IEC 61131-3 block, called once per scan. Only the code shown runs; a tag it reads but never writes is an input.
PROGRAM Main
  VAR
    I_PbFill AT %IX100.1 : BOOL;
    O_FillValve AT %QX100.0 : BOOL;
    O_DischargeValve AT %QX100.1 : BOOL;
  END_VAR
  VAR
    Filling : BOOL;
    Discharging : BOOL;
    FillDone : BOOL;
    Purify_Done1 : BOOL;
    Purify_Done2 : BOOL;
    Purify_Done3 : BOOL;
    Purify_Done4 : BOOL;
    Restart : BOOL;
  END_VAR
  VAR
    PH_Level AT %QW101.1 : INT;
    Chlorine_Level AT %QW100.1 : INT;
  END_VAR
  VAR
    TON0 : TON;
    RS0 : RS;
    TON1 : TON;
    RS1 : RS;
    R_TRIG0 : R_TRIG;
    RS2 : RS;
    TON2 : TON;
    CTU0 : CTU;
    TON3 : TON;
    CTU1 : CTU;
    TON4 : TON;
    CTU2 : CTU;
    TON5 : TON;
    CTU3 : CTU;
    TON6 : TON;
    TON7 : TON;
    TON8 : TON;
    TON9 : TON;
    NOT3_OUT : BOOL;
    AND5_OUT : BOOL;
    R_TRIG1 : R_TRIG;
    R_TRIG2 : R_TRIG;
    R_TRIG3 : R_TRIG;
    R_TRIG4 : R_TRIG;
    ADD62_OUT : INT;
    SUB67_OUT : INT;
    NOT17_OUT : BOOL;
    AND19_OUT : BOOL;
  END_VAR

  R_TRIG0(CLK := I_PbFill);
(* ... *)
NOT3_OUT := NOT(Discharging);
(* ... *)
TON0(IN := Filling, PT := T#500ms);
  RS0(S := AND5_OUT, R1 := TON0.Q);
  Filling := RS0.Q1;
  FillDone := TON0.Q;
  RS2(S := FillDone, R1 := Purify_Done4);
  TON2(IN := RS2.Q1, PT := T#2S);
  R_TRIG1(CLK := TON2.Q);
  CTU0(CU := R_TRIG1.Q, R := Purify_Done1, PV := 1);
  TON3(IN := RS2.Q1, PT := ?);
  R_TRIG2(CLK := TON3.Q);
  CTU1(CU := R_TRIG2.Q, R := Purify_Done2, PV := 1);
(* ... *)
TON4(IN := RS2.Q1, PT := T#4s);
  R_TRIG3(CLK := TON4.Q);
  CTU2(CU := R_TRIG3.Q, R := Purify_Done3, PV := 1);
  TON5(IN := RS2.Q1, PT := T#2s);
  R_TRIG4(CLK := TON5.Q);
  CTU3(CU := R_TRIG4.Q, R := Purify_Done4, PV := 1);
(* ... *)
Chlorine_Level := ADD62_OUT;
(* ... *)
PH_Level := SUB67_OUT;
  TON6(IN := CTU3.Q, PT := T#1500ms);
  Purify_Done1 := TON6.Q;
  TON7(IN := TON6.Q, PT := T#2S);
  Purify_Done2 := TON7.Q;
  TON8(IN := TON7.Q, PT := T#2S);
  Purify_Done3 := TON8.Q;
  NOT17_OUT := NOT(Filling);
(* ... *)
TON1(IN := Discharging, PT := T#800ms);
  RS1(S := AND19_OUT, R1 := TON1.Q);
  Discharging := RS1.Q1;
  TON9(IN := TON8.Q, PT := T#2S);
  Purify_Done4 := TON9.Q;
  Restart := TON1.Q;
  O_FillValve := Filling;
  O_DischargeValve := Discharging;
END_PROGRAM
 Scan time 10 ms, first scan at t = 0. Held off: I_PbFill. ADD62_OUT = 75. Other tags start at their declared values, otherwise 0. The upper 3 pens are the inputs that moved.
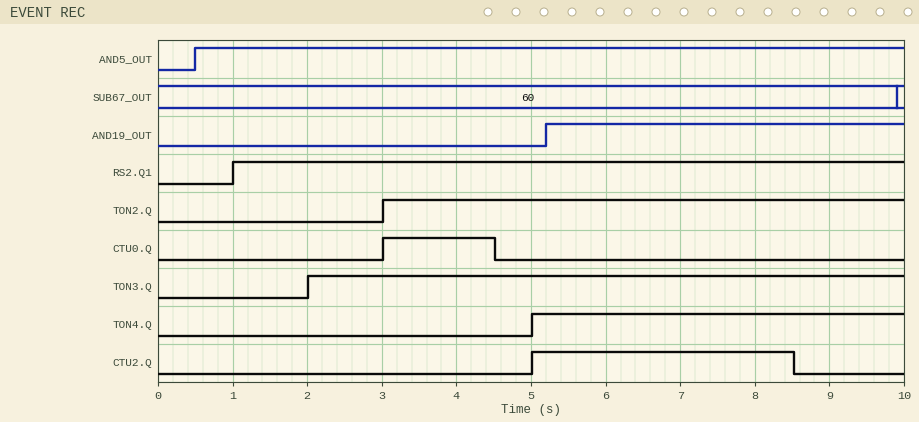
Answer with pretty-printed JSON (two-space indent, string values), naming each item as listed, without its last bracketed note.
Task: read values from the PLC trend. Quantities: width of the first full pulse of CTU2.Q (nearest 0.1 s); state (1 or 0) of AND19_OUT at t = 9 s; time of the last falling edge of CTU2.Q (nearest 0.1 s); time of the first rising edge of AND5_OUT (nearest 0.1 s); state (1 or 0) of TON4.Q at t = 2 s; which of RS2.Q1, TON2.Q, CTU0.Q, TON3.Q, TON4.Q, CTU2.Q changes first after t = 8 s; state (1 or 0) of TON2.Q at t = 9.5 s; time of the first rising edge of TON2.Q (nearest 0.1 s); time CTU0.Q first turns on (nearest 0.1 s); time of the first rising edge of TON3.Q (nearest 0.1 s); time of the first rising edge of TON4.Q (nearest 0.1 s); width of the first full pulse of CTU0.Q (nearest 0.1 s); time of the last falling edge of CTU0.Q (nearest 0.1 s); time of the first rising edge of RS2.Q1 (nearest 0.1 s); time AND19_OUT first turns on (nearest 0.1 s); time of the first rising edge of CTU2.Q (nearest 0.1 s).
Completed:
{
  "width of the first full pulse of CTU2.Q": "3.5 s",
  "state (1 or 0) of AND19_OUT at t = 9 s": "1",
  "time of the last falling edge of CTU2.Q": "8.5 s",
  "time of the first rising edge of AND5_OUT": "0.5 s",
  "state (1 or 0) of TON4.Q at t = 2 s": "0",
  "which of RS2.Q1, TON2.Q, CTU0.Q, TON3.Q, TON4.Q, CTU2.Q changes first after t = 8 s": "CTU2.Q",
  "state (1 or 0) of TON2.Q at t = 9.5 s": "1",
  "time of the first rising edge of TON2.Q": "3.0 s",
  "time CTU0.Q first turns on": "3.0 s",
  "time of the first rising edge of TON3.Q": "2.0 s",
  "time of the first rising edge of TON4.Q": "5.0 s",
  "width of the first full pulse of CTU0.Q": "1.5 s",
  "time of the last falling edge of CTU0.Q": "4.5 s",
  "time of the first rising edge of RS2.Q1": "1.0 s",
  "time AND19_OUT first turns on": "5.2 s",
  "time of the first rising edge of CTU2.Q": "5.0 s"
}
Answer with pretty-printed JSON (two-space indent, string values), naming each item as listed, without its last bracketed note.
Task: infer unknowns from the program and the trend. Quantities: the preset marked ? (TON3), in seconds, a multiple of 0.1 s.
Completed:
{
  "the preset marked ? (TON3), in seconds, a multiple of 0.1 s": "1.0 s"
}
